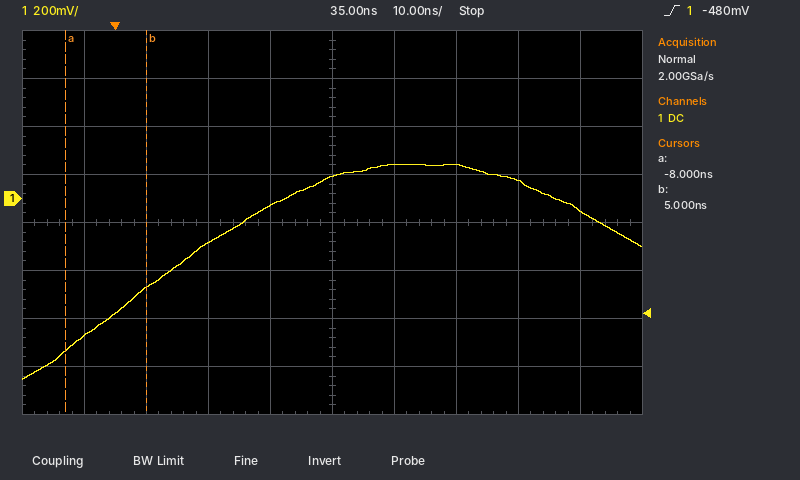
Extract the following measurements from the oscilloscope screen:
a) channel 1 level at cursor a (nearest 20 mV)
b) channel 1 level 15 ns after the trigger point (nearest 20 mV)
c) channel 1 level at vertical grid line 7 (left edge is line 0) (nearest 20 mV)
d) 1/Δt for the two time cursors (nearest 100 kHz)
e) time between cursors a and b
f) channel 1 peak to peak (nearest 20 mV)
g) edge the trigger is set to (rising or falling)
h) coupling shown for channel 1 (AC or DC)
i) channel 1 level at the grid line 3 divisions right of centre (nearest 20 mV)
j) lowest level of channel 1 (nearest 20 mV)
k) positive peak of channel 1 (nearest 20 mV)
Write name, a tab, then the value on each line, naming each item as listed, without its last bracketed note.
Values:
channel 1 level at cursor a	-640 mV
channel 1 level 15 ns after the trigger point	-180 mV
channel 1 level at vertical grid line 7 (left edge is line 0)	140 mV
1/Δt for the two time cursors	76.9 MHz
time between cursors a and b	13 ns
channel 1 peak to peak	900 mV
edge the trigger is set to	rising
coupling shown for channel 1	DC
channel 1 level at the grid line 3 divisions right of centre	80 mV
lowest level of channel 1	-760 mV
positive peak of channel 1	140 mV
